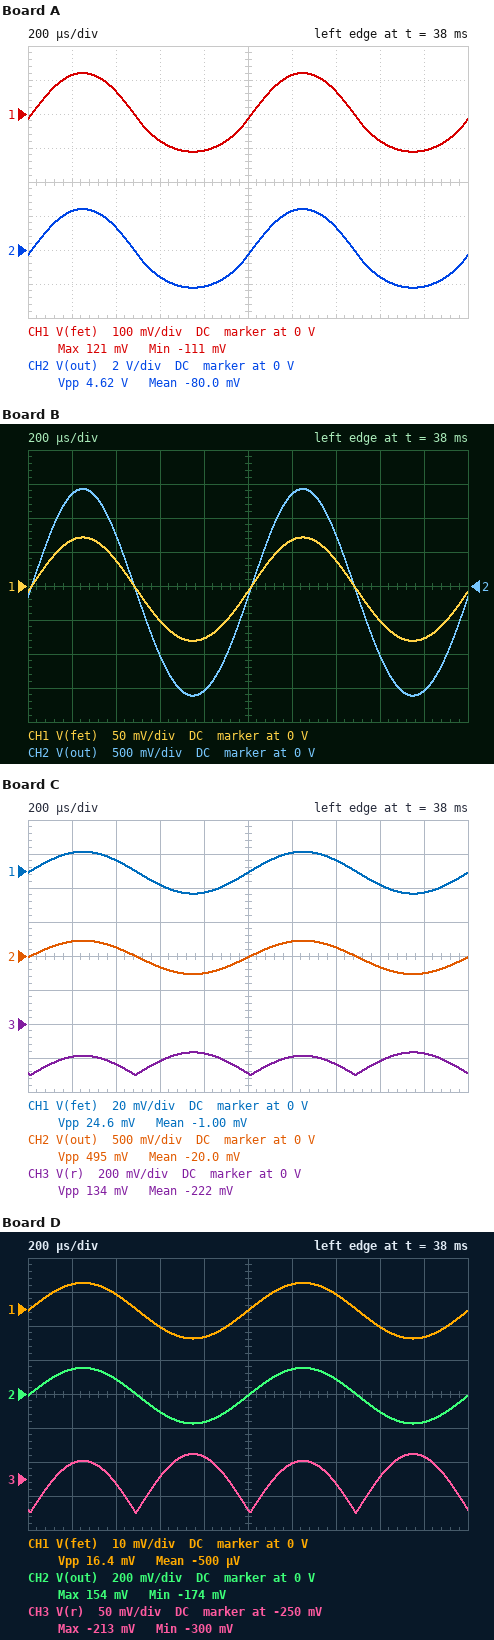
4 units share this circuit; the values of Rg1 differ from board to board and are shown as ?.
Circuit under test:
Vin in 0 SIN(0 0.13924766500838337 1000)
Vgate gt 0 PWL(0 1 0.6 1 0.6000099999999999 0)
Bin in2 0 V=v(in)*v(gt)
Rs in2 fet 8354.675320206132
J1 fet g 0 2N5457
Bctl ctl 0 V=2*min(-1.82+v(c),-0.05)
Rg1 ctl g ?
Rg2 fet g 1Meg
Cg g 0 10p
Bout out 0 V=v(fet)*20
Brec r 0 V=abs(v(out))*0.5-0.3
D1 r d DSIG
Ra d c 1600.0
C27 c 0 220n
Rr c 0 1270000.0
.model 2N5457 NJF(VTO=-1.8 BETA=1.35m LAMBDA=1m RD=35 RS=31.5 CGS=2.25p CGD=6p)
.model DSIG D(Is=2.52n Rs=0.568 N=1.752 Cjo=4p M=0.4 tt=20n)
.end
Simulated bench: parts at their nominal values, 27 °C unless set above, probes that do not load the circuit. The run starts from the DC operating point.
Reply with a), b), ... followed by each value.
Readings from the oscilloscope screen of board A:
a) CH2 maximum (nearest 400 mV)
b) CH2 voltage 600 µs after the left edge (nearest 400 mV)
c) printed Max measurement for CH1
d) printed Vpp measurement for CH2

a) 2.4 V
b) -1.6 V
c) 121 mV
d) 4.62 V
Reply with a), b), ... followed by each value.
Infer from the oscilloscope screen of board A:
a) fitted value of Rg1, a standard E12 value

a) 390 kΩ
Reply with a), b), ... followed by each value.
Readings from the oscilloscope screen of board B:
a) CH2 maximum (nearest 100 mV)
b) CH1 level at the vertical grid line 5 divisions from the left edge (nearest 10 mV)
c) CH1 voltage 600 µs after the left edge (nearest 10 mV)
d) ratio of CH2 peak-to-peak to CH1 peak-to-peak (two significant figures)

a) 1.4 V
b) -10 mV
c) -50 mV
d) 20
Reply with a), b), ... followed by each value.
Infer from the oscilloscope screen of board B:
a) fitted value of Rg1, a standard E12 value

a) 820 kΩ
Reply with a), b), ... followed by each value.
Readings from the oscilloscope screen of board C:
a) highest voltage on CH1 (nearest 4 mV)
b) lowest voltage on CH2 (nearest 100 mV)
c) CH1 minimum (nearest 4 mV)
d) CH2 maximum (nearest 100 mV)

a) 12 mV
b) -300 mV
c) -12 mV
d) 200 mV
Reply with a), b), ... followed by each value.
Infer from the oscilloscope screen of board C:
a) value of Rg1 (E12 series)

a) 1.8 MΩ
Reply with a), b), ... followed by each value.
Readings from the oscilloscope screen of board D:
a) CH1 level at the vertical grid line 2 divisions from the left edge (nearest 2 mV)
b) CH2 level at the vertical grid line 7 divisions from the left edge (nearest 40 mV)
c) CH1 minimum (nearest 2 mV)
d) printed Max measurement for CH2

a) 4 mV
b) 80 mV
c) -8 mV
d) 154 mV
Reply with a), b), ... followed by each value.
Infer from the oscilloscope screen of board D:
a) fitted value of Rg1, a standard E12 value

a) 2.7 MΩ
